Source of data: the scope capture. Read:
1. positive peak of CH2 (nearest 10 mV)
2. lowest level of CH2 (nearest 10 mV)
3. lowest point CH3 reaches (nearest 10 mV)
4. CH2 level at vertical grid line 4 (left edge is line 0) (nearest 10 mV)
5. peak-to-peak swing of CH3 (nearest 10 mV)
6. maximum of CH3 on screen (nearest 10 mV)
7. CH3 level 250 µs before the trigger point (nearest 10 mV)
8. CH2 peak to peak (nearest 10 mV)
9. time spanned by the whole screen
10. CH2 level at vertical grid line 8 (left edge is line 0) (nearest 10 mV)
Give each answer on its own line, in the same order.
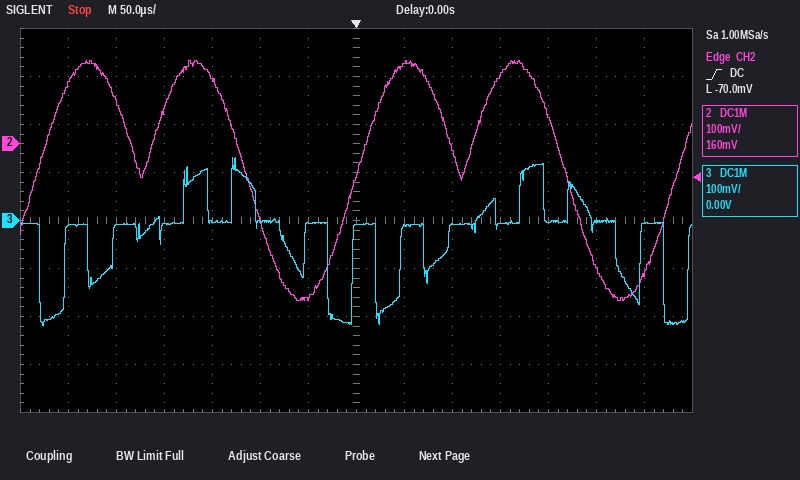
170 mV
-330 mV
-220 mV
140 mV
350 mV
130 mV
-10 mV
500 mV
700 µs
170 mV
